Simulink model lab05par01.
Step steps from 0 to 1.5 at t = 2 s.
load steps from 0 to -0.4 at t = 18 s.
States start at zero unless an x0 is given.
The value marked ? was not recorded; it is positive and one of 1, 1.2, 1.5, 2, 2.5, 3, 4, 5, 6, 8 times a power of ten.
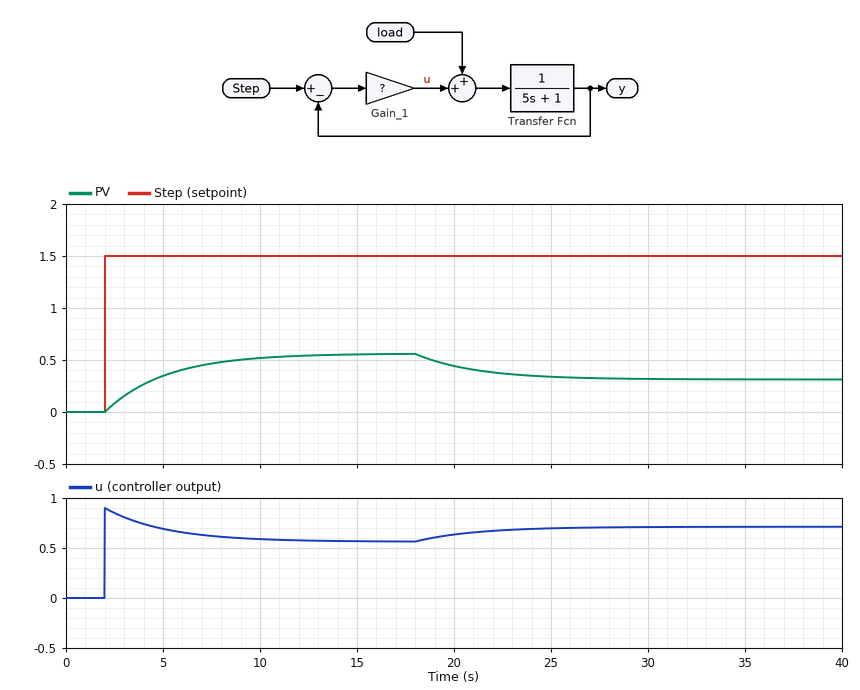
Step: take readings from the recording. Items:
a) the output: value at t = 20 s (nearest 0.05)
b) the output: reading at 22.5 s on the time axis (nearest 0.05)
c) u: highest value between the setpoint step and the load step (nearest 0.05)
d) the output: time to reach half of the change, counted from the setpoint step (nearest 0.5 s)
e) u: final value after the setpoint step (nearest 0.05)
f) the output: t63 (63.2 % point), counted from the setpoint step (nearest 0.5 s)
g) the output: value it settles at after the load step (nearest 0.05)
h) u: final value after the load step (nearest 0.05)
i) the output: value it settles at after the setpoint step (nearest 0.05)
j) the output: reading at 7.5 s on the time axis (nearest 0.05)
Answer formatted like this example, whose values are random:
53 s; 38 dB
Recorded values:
0.45; 0.35; 0.90; 2.0 s; 0.55; 3.0 s; 0.30; 0.70; 0.55; 0.45
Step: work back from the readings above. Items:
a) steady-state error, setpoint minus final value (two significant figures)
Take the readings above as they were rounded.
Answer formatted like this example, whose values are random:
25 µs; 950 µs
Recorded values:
0.95
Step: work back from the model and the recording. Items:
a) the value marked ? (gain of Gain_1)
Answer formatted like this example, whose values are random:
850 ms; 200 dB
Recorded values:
0.6
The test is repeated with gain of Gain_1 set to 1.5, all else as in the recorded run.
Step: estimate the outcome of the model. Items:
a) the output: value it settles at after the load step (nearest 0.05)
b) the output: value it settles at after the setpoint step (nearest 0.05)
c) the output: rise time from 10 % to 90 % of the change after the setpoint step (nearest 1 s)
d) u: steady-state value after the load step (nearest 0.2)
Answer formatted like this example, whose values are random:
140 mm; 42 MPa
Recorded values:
0.75; 0.90; 4 s; 1.2
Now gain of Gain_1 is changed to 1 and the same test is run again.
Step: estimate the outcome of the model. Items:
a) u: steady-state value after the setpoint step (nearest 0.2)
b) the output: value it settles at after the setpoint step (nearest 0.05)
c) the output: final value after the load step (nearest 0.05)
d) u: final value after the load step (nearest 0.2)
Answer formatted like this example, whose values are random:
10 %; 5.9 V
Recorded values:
0.8; 0.75; 0.55; 1.0
